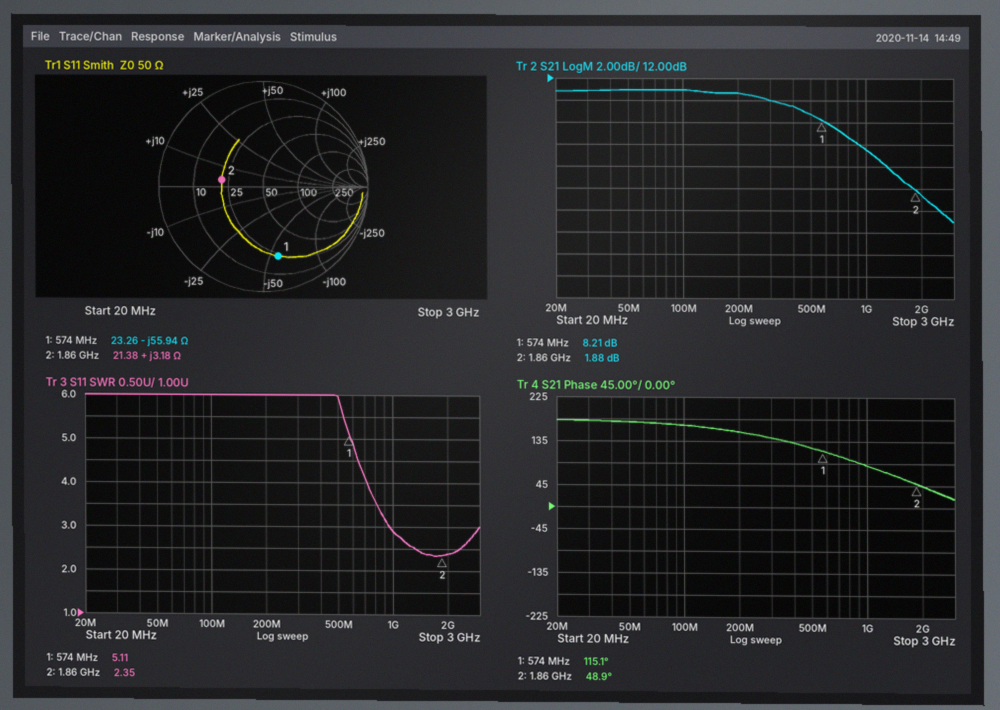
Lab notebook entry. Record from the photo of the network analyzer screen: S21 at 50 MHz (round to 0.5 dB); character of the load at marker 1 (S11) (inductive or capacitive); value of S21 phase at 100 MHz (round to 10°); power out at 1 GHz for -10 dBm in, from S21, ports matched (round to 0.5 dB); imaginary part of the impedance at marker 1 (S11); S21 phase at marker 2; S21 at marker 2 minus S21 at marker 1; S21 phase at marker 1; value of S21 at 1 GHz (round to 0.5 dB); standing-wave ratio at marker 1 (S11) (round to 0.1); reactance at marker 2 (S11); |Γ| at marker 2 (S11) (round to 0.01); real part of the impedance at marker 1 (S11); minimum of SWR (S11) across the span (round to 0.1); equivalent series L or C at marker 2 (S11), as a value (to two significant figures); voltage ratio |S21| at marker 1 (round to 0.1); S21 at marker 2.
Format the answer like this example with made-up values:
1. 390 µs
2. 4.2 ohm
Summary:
1. 11.0 dB
2. capacitive
3. 170°
4. -4.5 dBm
5. -55.94 Ω
6. 48.9°
7. -6.33 dB
8. 115.1°
9. 5.5 dB
10. 5.1
11. +3.18 Ω
12. 0.40
13. 23.26 Ω
14. 2.3
15. 270 pH
16. 2.6
17. 1.88 dB
